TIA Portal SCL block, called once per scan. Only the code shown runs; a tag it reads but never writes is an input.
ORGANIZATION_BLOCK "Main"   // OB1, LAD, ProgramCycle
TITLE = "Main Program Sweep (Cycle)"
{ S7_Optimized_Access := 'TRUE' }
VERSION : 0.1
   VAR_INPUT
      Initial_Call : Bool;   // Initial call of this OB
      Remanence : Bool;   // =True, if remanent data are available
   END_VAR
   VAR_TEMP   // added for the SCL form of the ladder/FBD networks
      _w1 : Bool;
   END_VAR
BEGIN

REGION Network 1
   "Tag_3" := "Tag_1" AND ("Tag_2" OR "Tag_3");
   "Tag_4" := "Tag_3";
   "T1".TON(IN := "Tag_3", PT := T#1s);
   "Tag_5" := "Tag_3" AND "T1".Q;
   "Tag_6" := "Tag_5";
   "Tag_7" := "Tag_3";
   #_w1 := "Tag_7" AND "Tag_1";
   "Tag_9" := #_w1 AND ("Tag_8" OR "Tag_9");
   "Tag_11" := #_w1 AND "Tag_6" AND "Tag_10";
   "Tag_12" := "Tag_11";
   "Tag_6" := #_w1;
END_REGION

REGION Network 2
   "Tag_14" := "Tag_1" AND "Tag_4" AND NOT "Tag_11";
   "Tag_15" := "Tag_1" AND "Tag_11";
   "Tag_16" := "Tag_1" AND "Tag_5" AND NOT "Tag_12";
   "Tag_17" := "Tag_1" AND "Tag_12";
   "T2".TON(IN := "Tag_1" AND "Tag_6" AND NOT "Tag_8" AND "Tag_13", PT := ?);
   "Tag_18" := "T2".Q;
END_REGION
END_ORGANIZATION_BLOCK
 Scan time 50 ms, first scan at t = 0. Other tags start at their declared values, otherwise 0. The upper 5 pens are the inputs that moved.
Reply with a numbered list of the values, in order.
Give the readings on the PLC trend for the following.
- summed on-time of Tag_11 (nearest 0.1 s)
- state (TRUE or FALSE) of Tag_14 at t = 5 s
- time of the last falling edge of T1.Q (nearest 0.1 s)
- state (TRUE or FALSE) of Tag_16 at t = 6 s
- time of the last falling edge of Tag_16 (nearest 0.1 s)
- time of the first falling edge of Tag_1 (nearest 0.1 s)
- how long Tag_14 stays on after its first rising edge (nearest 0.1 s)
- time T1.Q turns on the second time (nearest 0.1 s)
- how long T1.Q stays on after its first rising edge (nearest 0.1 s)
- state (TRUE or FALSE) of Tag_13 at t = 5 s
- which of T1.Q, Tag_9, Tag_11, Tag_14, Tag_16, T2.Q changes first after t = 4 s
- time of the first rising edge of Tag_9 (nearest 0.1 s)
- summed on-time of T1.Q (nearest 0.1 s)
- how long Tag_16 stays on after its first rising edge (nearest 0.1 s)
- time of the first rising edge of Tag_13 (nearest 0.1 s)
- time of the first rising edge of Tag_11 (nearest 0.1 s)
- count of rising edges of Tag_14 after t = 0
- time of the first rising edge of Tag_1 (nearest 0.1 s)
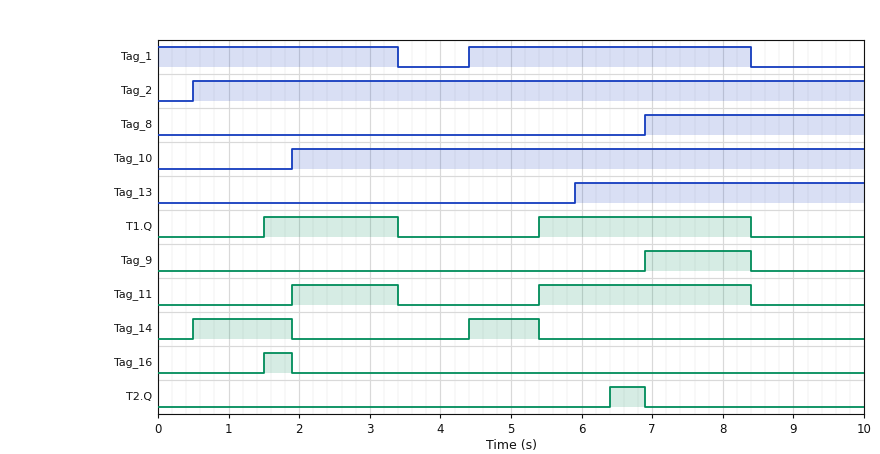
1. 4.5 s
2. TRUE
3. 8.4 s
4. FALSE
5. 1.9 s
6. 3.4 s
7. 1.4 s
8. 5.4 s
9. 1.9 s
10. FALSE
11. Tag_14
12. 6.9 s
13. 4.9 s
14. 0.4 s
15. 5.9 s
16. 1.9 s
17. 2
18. 4.4 s
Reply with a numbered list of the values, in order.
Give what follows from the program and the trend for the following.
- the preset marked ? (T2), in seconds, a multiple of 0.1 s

1. 0.5 s
